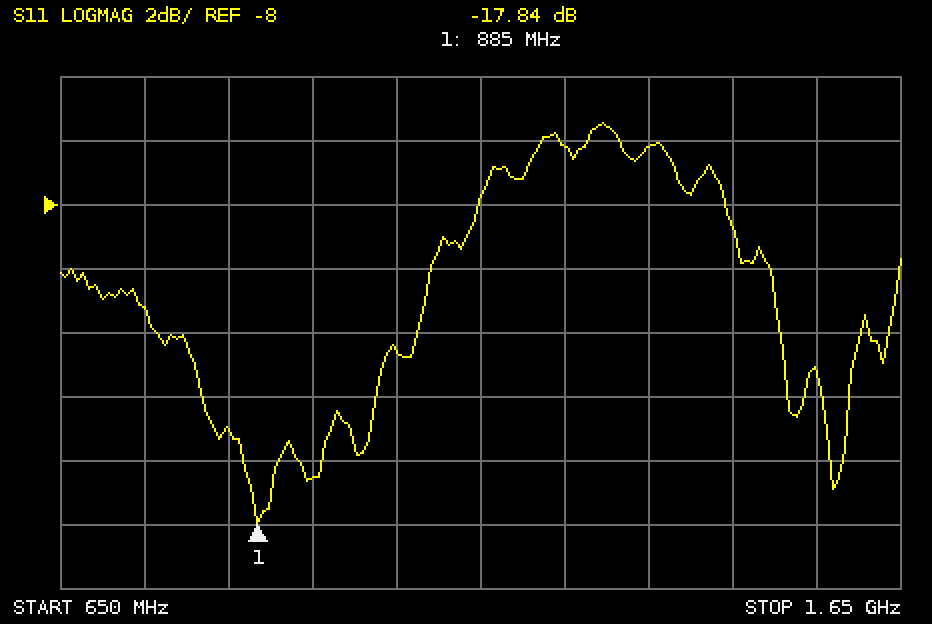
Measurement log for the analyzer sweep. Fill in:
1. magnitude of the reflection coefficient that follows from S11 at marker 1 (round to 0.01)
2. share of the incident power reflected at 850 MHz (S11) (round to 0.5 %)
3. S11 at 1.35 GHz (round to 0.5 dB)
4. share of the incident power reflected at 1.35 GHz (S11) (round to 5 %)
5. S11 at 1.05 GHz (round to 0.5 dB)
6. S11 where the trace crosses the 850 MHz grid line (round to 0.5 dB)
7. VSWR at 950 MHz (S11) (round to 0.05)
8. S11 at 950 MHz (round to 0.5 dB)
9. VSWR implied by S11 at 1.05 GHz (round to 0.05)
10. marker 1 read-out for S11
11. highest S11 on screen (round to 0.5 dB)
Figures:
0.13
3.0 %
-6.0 dB
25 %
-12.5 dB
-15.0 dB
1.35
-16.5 dB
1.60
-17.84 dB
-5.5 dB
